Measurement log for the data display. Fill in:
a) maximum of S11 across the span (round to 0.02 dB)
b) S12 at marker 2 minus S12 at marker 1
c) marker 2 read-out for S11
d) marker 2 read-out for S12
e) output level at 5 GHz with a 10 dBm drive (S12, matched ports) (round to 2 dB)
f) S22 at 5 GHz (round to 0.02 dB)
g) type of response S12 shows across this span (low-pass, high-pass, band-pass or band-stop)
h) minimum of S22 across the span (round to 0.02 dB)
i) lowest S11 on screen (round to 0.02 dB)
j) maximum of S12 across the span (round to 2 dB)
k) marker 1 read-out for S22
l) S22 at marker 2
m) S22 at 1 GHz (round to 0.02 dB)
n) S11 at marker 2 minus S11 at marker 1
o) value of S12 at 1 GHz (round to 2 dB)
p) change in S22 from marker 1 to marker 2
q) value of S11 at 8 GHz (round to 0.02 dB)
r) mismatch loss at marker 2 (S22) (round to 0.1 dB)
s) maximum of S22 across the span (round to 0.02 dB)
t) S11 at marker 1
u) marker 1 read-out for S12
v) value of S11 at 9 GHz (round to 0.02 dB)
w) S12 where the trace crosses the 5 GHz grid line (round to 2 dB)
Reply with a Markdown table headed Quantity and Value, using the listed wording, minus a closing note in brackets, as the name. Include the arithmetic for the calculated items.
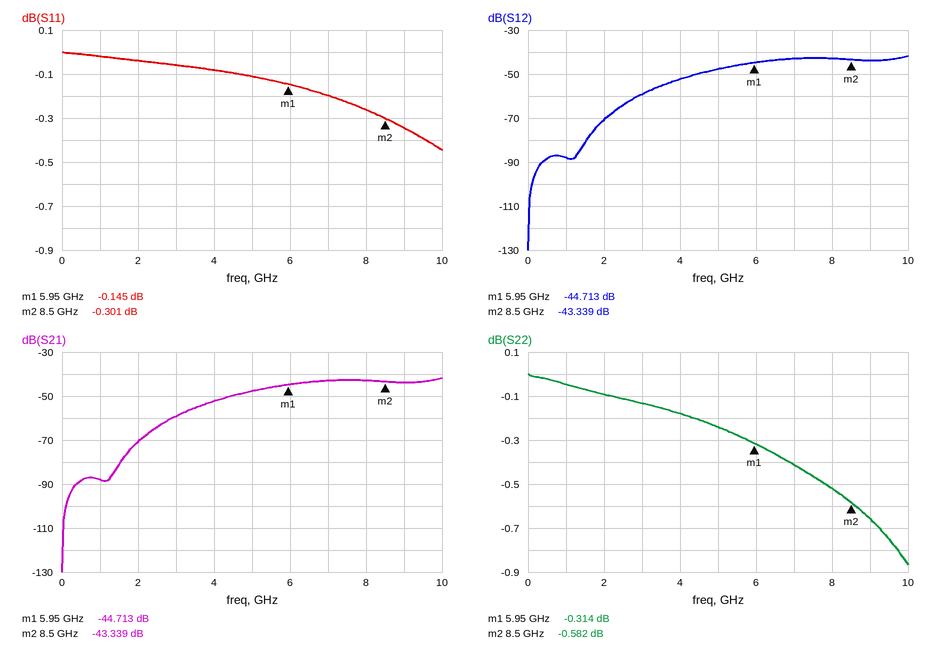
| Quantity | Value |
|---|---|
| maximum of S11 across the span | 0.00 dB |
| S12 at marker 2 minus S12 at marker 1 | -43.339 − (-44.713) = 1.374 dB |
| marker 2 read-out for S11 | -0.301 dB |
| marker 2 read-out for S12 | -43.339 dB |
| output level at 5 GHz with a 10 dBm drive (S12, matched ports) | 10 dBm + (-48 dB) = -38 dBm |
| S22 at 5 GHz | -0.24 dB |
| type of response S12 shows across this span | high-pass |
| minimum of S22 across the span | -0.86 dB |
| lowest S11 on screen | -0.44 dB |
| maximum of S12 across the span | -42 dB |
| marker 1 read-out for S22 | -0.314 dB |
| S22 at marker 2 | -0.582 dB |
| S22 at 1 GHz | -0.04 dB |
| S11 at marker 2 minus S11 at marker 1 | -0.301 − (-0.145) = -0.156 dB |
| value of S12 at 1 GHz | -88 dB |
| change in S22 from marker 1 to marker 2 | -0.582 − (-0.314) = -0.268 dB |
| value of S11 at 8 GHz | -0.26 dB |
| mismatch loss at marker 2 (S22) | −10 log10(1 − 10^(-0.582/10)) ≈ 9.0 dB |
| maximum of S22 across the span | 0.00 dB |
| S11 at marker 1 | -0.145 dB |
| marker 1 read-out for S12 | -44.713 dB |
| value of S11 at 9 GHz | -0.34 dB |
| S12 where the trace crosses the 5 GHz grid line | -48 dB |
